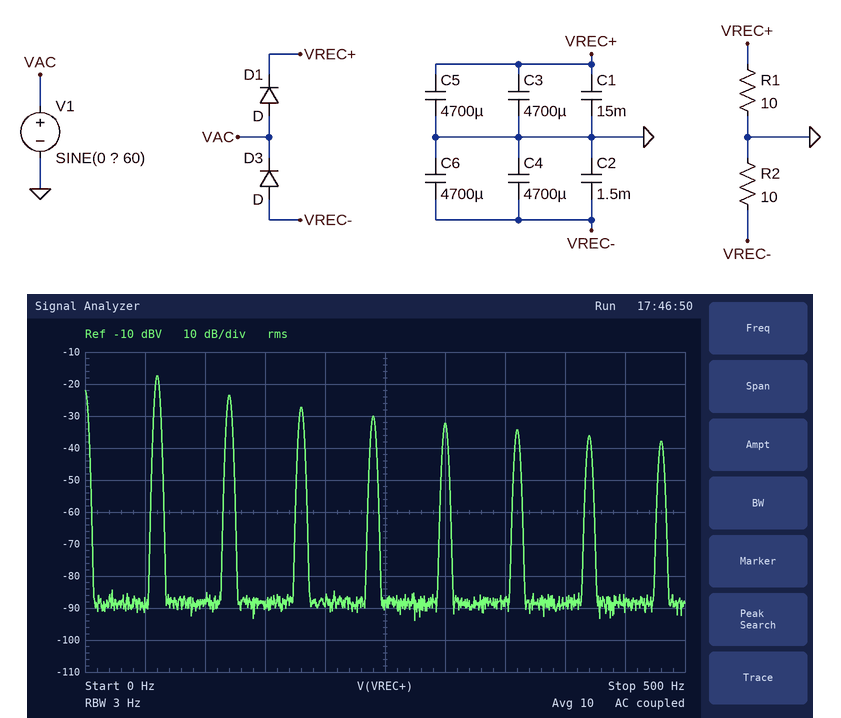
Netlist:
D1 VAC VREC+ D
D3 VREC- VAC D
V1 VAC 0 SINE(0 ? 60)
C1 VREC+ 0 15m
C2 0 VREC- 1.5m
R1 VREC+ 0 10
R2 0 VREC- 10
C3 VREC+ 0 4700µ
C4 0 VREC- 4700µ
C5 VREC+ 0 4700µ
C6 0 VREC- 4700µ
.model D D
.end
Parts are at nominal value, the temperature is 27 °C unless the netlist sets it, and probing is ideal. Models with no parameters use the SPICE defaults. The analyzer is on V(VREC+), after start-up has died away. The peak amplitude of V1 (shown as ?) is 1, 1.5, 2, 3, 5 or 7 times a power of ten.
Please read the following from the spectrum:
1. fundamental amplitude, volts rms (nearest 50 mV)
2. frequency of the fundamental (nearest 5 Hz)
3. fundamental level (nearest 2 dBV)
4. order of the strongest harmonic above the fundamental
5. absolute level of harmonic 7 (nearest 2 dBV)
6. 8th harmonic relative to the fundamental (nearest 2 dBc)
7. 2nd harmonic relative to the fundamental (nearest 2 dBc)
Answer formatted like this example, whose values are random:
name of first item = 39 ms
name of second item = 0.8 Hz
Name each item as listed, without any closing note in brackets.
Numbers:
fundamental amplitude, volts rms = 150 mV
frequency of the fundamental = 60 Hz
fundamental level = -18 dBV
order of the strongest harmonic above the fundamental = 2
absolute level of harmonic 7 = -36 dBV
8th harmonic relative to the fundamental = -20 dBc
2nd harmonic relative to the fundamental = -6 dBc
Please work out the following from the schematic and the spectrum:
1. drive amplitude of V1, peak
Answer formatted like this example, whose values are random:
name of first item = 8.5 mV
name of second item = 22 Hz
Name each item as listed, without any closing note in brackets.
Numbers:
drive amplitude of V1, peak = 10 V
